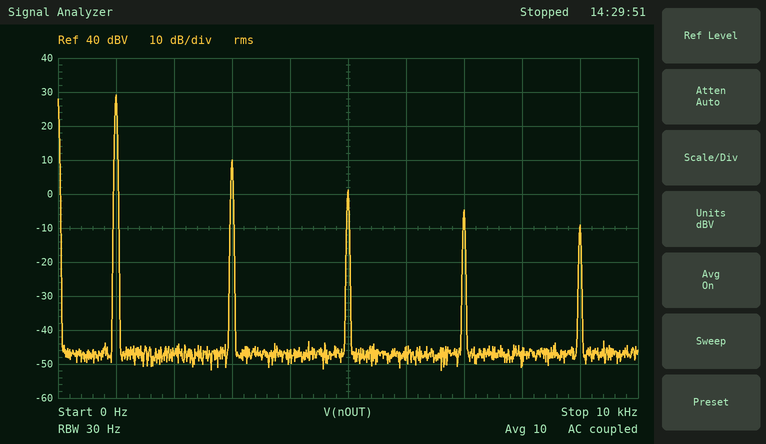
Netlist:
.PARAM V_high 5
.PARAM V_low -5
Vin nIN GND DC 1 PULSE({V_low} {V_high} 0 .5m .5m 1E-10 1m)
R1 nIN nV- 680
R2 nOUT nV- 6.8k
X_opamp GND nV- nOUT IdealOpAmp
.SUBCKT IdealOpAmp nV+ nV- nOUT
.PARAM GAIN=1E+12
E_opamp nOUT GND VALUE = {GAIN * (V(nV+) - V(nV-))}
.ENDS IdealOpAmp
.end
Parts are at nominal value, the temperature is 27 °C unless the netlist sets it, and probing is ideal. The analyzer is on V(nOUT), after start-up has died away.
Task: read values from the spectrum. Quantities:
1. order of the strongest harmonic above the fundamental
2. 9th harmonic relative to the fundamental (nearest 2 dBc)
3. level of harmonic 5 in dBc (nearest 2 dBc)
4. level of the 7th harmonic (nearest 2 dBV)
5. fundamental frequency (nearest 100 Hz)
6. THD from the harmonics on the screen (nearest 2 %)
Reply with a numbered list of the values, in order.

1. 3
2. -38 dBc
3. -28 dBc
4. -4 dBV
5. 1.0 kHz
6. 12 %
